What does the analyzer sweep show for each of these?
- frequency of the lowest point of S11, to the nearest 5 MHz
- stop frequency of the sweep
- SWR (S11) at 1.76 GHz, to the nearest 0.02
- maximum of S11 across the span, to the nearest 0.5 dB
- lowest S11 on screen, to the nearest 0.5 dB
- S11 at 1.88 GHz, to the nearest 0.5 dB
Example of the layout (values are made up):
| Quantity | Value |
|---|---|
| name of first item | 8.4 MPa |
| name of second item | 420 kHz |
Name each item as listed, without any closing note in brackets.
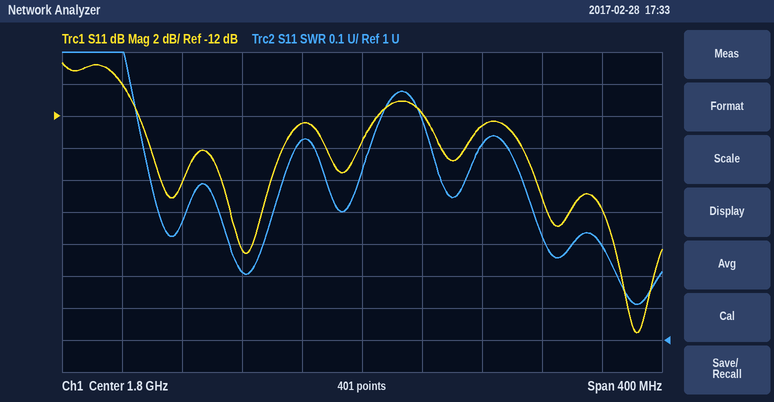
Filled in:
| Quantity | Value |
|---|---|
| frequency of the lowest point of S11, to the nearest 5 MHz | 1.985 GHz |
| stop frequency of the sweep | 2 GHz |
| SWR (S11) at 1.76 GHz, to the nearest 0.02 | 1.62 |
| maximum of S11 across the span, to the nearest 0.5 dB | -8.5 dB |
| lowest S11 on screen, to the nearest 0.5 dB | -25.5 dB |
| S11 at 1.88 GHz, to the nearest 0.5 dB | -12.5 dB |
